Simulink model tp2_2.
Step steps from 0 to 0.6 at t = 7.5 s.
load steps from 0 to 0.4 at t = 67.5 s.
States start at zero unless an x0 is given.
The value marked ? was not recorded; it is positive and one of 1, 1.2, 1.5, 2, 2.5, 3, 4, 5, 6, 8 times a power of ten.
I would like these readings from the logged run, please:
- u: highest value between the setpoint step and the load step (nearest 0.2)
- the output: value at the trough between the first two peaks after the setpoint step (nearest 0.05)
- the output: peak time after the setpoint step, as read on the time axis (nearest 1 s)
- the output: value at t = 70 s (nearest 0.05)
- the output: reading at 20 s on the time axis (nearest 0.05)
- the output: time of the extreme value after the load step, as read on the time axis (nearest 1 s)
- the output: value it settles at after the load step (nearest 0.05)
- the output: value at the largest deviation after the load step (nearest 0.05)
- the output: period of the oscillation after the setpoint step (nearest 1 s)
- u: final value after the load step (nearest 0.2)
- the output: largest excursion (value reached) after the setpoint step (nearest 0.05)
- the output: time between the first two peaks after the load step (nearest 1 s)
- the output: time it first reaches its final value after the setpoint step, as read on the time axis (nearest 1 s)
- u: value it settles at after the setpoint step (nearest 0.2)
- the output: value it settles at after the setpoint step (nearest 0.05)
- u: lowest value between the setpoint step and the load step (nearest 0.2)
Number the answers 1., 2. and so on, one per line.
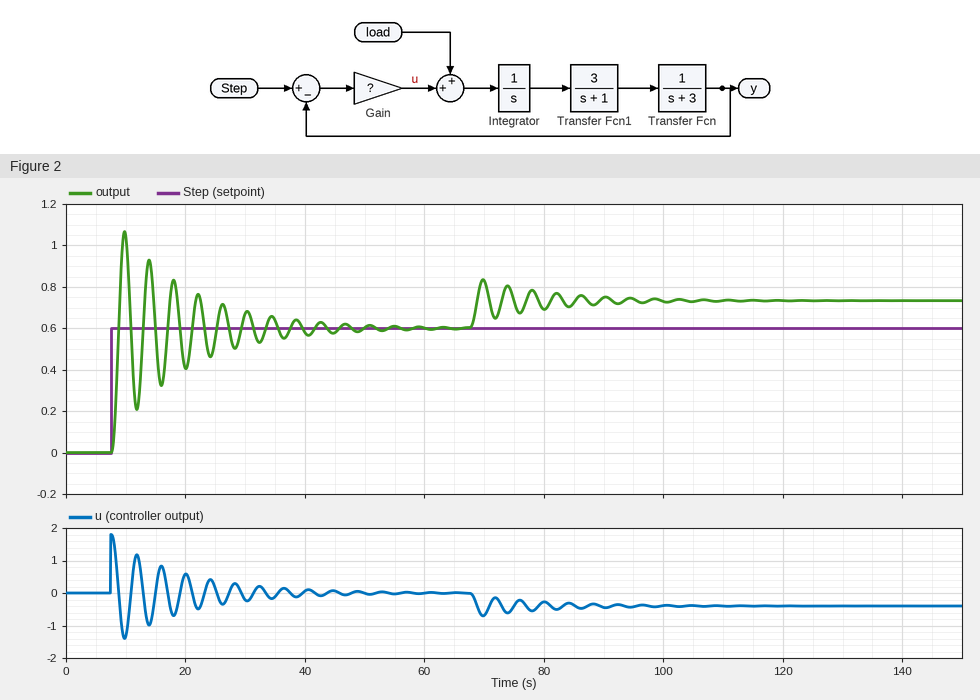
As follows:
1. 1.8
2. 0.20
3. 10 s
4. 0.85
5. 0.40
6. 70 s
7. 0.75
8. 0.85
9. 4 s
10. -0.4
11. 1.05
12. 4 s
13. 9 s
14. 0.0
15. 0.60
16. -1.4
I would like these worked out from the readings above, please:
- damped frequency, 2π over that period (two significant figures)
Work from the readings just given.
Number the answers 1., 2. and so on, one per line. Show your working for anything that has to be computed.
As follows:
1. 2π / 4 = 1.6 rad/s
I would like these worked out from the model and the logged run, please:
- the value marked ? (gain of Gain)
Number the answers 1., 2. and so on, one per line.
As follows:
1. 3
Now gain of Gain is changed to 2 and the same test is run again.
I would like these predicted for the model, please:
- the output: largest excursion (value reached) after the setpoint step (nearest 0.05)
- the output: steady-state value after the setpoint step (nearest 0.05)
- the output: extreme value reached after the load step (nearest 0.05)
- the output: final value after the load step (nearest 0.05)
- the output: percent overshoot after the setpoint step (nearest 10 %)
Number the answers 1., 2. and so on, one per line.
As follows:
1. 0.95
2. 0.60
3. 0.90
4. 0.80
5. 60 %
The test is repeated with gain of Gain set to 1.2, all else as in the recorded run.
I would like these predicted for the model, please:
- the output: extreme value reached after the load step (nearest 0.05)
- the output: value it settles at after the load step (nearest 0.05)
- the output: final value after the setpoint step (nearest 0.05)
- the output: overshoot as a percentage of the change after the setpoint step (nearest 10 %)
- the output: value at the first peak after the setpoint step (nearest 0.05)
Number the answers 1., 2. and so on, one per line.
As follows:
1. 1.05
2. 0.95
3. 0.60
4. 40 %
5. 0.85
